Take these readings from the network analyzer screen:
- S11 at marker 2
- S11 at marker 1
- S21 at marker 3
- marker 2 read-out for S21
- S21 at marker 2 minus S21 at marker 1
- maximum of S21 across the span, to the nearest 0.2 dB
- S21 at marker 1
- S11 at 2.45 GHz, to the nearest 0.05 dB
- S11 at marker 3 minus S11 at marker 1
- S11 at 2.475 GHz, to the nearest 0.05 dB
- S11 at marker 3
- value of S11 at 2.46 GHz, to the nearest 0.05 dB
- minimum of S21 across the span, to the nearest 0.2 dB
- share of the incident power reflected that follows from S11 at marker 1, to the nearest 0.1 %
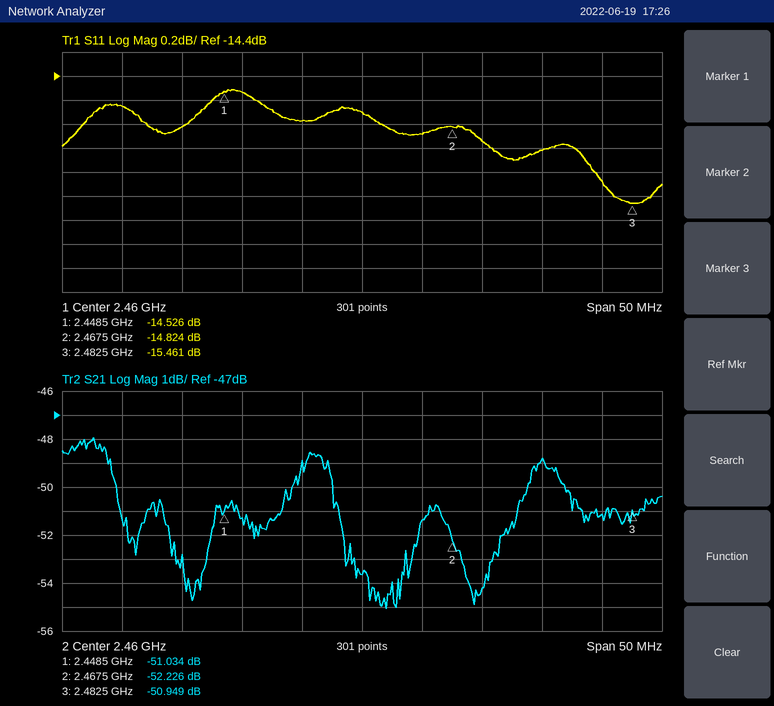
-14.824 dB
-14.526 dB
-50.949 dB
-52.226 dB
-1.192 dB
-48.0 dB
-51.034 dB
-14.55 dB
-0.935 dB
-15.00 dB
-15.461 dB
-14.70 dB
-55.0 dB
3.5 %
